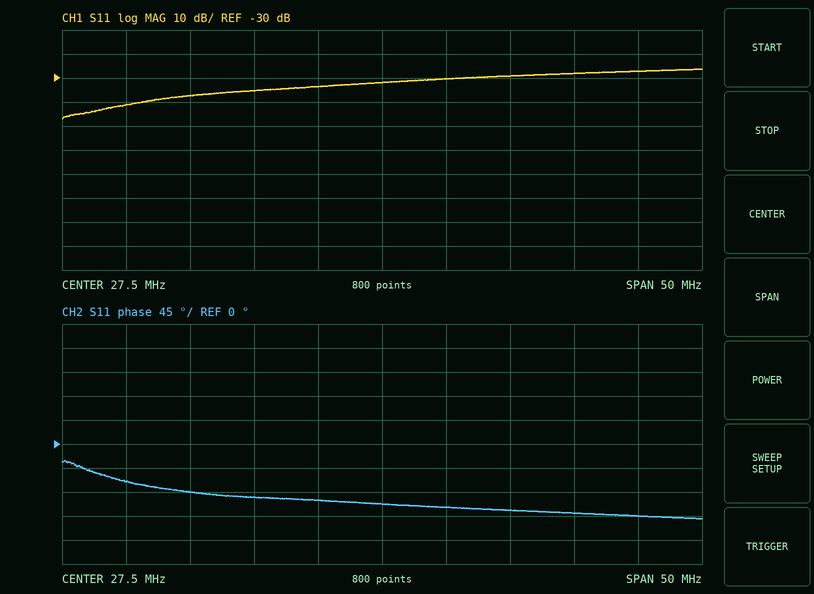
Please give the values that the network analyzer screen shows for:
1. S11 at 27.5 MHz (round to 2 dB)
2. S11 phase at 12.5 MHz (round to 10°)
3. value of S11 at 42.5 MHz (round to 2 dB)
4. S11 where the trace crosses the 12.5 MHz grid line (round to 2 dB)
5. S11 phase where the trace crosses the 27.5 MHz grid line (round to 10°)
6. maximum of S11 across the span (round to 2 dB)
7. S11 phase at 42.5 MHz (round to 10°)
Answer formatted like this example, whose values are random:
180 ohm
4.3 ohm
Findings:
-32 dB
-90°
-28 dB
-38 dB
-110°
-26 dB
-130°
